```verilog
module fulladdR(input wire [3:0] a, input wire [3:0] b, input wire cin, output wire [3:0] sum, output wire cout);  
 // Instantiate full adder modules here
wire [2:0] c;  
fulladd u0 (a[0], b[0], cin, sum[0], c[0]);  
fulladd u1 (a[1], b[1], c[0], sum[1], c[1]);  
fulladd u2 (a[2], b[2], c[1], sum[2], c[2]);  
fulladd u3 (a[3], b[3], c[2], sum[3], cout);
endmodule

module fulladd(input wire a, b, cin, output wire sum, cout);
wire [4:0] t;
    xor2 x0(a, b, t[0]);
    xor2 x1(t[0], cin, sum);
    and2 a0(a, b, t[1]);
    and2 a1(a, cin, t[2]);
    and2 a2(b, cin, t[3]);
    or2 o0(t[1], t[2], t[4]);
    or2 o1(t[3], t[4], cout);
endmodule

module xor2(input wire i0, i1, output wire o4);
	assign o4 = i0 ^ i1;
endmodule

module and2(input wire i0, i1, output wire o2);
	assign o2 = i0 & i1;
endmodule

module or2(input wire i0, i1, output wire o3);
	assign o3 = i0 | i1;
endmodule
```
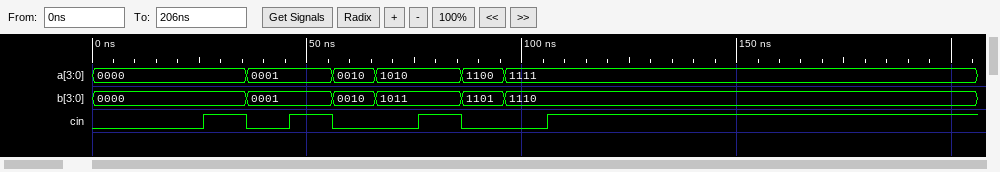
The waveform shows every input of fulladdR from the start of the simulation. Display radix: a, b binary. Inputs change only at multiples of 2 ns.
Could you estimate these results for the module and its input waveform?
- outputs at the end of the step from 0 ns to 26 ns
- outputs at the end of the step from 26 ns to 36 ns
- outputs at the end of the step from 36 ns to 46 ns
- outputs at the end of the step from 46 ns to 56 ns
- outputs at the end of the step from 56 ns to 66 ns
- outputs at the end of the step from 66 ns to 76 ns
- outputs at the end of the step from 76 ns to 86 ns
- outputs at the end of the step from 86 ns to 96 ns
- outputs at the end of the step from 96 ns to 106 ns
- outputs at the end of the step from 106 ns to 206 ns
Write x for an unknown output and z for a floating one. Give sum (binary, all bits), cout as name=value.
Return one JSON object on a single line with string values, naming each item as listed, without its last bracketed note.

{"outputs at the end of the step from 0 ns to 26 ns": "sum=0000, cout=0", "outputs at the end of the step from 26 ns to 36 ns": "sum=0001, cout=0", "outputs at the end of the step from 36 ns to 46 ns": "sum=0010, cout=0", "outputs at the end of the step from 46 ns to 56 ns": "sum=0011, cout=0", "outputs at the end of the step from 56 ns to 66 ns": "sum=0100, cout=0", "outputs at the end of the step from 66 ns to 76 ns": "sum=0101, cout=1", "outputs at the end of the step from 76 ns to 86 ns": "sum=0110, cout=1", "outputs at the end of the step from 86 ns to 96 ns": "sum=1001, cout=1", "outputs at the end of the step from 96 ns to 106 ns": "sum=1101, cout=1", "outputs at the end of the step from 106 ns to 206 ns": "sum=1110, cout=1"}
